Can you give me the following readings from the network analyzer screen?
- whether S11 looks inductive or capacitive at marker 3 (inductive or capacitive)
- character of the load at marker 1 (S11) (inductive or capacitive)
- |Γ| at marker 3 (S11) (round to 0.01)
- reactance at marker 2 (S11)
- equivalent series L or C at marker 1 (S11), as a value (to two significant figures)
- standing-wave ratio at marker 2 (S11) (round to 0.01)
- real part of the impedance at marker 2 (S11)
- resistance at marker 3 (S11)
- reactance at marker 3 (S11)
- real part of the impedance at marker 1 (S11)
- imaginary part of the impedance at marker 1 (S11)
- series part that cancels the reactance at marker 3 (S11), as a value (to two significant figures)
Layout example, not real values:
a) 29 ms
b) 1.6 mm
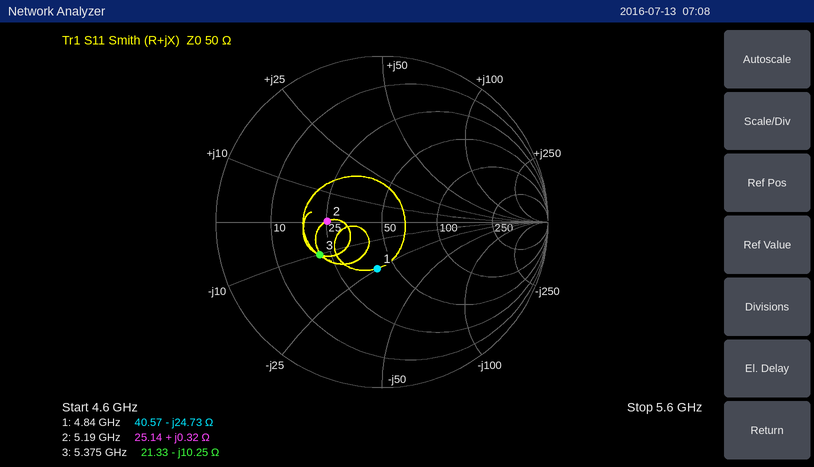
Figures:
a) capacitive
b) capacitive
c) 0.42
d) +0.32 Ω
e) 1.3 pF
f) 1.99
g) 25.14 Ω
h) 21.33 Ω
i) -10.25 Ω
j) 40.57 Ω
k) -24.73 Ω
l) 300 pH
